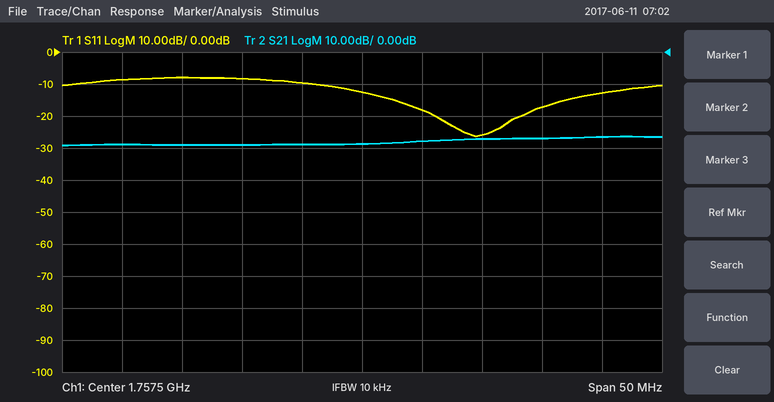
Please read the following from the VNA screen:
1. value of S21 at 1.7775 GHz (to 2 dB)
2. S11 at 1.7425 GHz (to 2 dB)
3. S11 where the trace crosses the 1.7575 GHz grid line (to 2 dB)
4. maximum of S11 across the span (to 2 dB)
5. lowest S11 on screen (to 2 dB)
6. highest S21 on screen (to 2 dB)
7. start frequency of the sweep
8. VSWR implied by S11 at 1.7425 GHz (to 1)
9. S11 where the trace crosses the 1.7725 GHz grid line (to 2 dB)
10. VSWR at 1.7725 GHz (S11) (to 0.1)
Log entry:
-26 dB
-8 dB
-12 dB
-8 dB
-26 dB
-26 dB
1.7325 GHz
2
-18 dB
1.3
